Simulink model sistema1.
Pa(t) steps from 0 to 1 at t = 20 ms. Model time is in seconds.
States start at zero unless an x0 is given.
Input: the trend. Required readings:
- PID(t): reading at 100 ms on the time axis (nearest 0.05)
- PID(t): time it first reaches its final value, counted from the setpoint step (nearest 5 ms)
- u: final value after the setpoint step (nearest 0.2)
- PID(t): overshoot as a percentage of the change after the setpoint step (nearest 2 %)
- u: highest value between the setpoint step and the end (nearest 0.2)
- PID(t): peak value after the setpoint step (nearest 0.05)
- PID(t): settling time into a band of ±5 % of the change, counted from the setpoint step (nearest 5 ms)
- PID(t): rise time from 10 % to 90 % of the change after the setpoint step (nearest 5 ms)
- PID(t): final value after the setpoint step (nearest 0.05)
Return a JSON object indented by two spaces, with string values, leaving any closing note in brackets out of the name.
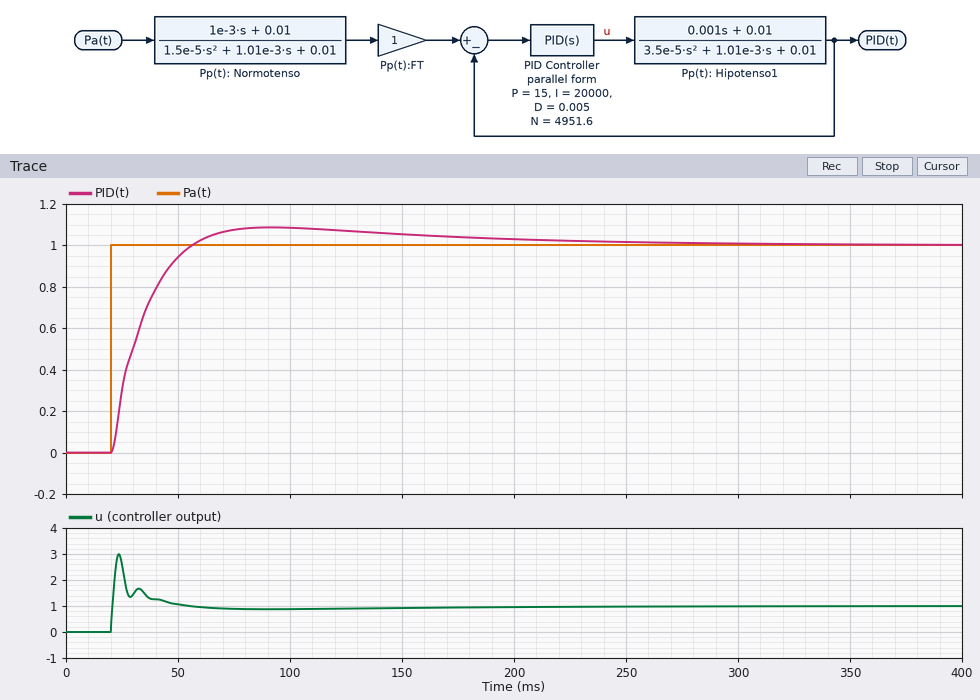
{
  "PID(t): reading at 100 ms on the time axis": "1.10",
  "PID(t): time it first reaches its final value, counted from the setpoint step": "35 ms",
  "u: final value after the setpoint step": "1.0",
  "PID(t): overshoot as a percentage of the change after the setpoint step": "8 %",
  "u: highest value between the setpoint step and the end": "3.0",
  "PID(t): peak value after the setpoint step": "1.10",
  "PID(t): settling time into a band of ±5 % of the change, counted from the setpoint step": "135 ms",
  "PID(t): rise time from 10 % to 90 % of the change after the setpoint step": "25 ms",
  "PID(t): final value after the setpoint step": "1.00"
}
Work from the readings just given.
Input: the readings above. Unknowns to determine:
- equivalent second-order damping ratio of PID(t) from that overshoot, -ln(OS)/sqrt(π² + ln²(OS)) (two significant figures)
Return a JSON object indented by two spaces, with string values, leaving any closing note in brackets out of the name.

{
  "equivalent second-order damping ratio of PID(t) from that overshoot, -ln(OS)/sqrt(π² + ln²(OS))": "0.63"
}
